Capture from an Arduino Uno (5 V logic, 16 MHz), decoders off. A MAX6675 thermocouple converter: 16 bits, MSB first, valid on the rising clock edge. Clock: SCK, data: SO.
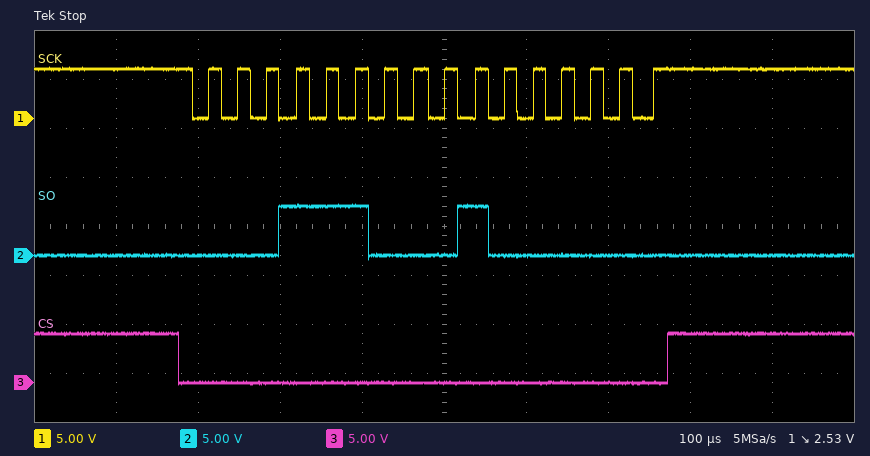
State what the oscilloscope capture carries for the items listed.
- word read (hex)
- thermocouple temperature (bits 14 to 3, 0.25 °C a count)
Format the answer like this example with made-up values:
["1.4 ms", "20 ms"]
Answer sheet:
["0x1C40", "226.00 °C"]
